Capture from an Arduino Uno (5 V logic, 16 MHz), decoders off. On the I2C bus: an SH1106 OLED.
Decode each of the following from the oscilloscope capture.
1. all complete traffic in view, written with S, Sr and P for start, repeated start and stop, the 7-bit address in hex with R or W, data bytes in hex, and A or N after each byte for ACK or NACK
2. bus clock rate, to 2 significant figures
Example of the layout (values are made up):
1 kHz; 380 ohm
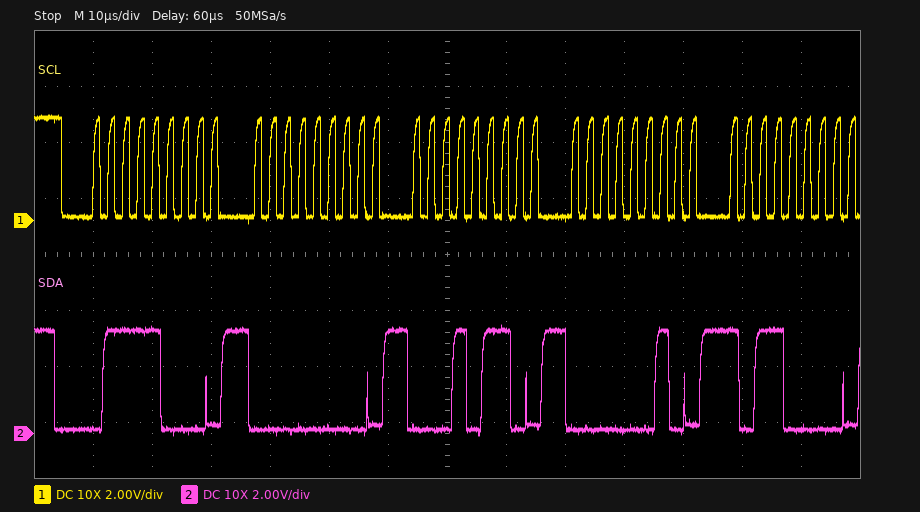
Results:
S 3CW A 00 A 16 A 02 A B0 A; 400 kHz
